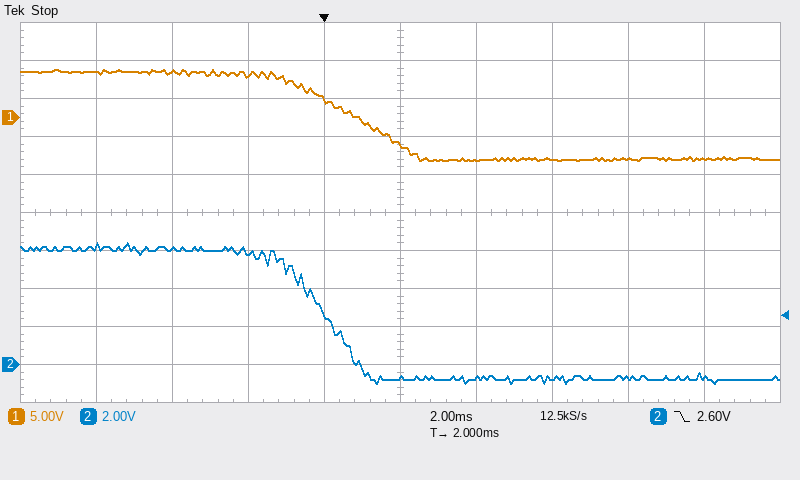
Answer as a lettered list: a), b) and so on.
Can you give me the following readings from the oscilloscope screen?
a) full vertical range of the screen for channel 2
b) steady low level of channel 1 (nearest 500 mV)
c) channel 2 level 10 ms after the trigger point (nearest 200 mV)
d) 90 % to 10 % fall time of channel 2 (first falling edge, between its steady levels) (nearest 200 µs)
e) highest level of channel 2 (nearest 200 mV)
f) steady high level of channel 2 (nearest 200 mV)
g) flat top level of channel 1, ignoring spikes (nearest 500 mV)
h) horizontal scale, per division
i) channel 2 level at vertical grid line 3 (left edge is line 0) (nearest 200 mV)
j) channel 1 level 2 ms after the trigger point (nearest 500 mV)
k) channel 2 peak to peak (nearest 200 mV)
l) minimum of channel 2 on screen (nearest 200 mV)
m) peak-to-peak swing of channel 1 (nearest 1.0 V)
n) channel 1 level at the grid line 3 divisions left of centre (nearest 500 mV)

a) 20 V
b) -5.5 V
c) -600 mV
d) 2.0 ms
e) 6.4 V
f) 6.0 V
g) 6.0 V
h) 2 ms
i) 6.0 V
j) -3.5 V
k) 7.4 V
l) -1.0 V
m) 12.0 V
n) 6.0 V
